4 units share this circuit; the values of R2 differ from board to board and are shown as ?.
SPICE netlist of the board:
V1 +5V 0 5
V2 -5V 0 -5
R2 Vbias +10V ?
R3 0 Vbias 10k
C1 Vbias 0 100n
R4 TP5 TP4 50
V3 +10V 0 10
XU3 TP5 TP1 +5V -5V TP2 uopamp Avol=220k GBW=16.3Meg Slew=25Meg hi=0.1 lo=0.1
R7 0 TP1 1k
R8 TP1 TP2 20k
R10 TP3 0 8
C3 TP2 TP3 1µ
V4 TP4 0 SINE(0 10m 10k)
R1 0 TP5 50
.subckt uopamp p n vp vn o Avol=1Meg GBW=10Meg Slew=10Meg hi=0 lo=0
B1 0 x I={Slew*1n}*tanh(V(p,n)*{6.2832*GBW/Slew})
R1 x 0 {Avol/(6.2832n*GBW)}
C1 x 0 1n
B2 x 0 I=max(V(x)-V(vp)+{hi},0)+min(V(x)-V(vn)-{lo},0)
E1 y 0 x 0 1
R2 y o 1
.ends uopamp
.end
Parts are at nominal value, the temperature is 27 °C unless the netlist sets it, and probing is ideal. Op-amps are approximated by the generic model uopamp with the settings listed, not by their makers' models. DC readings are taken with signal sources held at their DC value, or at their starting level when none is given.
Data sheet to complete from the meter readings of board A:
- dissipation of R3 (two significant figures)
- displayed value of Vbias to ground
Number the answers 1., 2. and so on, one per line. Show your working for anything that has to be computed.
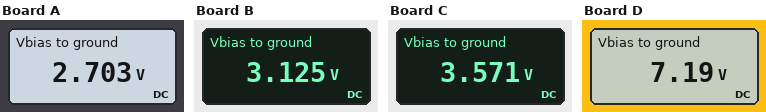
1. (2.703 V)^2 / 10 kΩ = 730 µW
2. 2.703 V
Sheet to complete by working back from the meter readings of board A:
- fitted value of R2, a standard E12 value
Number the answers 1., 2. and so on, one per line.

1. 27 kΩ
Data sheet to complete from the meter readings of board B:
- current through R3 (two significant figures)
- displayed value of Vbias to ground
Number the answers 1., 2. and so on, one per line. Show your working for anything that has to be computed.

1. (3.125 V) / 10 kΩ = 310 µA
2. 3.125 V
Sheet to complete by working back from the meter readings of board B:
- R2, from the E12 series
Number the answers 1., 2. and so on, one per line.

1. 22 kΩ
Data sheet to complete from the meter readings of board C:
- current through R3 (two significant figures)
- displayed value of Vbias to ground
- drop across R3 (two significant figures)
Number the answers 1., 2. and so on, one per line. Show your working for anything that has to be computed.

1. (3.571 V) / 10 kΩ = 360 µA
2. 3.571 V
3. 3.571 V = 3.6 V
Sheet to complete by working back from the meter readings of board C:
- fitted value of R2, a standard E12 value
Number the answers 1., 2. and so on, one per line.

1. 18 kΩ
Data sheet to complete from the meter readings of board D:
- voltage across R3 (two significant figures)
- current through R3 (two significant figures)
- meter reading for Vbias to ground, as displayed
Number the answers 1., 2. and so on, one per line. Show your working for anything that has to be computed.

1. 7.19 V = 7.2 V
2. (7.19 V) / 10 kΩ = 720 µA
3. 7.19 V
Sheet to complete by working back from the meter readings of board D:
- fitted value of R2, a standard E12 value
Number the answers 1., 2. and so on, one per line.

1. 3.9 kΩ
